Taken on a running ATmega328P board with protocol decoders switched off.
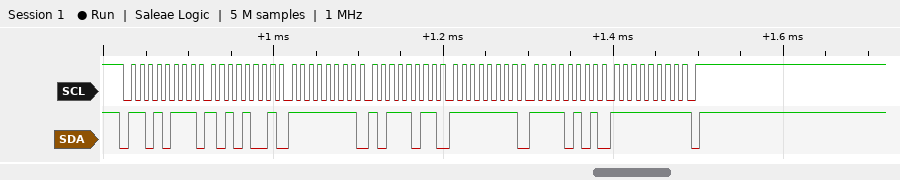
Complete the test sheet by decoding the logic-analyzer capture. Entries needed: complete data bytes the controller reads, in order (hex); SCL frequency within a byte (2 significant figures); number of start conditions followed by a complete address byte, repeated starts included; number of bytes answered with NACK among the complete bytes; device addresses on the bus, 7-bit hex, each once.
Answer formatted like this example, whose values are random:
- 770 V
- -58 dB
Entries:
- A9 FF BB FF F5 FF
- 100 kHz
- 1
- 1
- 0x6B
